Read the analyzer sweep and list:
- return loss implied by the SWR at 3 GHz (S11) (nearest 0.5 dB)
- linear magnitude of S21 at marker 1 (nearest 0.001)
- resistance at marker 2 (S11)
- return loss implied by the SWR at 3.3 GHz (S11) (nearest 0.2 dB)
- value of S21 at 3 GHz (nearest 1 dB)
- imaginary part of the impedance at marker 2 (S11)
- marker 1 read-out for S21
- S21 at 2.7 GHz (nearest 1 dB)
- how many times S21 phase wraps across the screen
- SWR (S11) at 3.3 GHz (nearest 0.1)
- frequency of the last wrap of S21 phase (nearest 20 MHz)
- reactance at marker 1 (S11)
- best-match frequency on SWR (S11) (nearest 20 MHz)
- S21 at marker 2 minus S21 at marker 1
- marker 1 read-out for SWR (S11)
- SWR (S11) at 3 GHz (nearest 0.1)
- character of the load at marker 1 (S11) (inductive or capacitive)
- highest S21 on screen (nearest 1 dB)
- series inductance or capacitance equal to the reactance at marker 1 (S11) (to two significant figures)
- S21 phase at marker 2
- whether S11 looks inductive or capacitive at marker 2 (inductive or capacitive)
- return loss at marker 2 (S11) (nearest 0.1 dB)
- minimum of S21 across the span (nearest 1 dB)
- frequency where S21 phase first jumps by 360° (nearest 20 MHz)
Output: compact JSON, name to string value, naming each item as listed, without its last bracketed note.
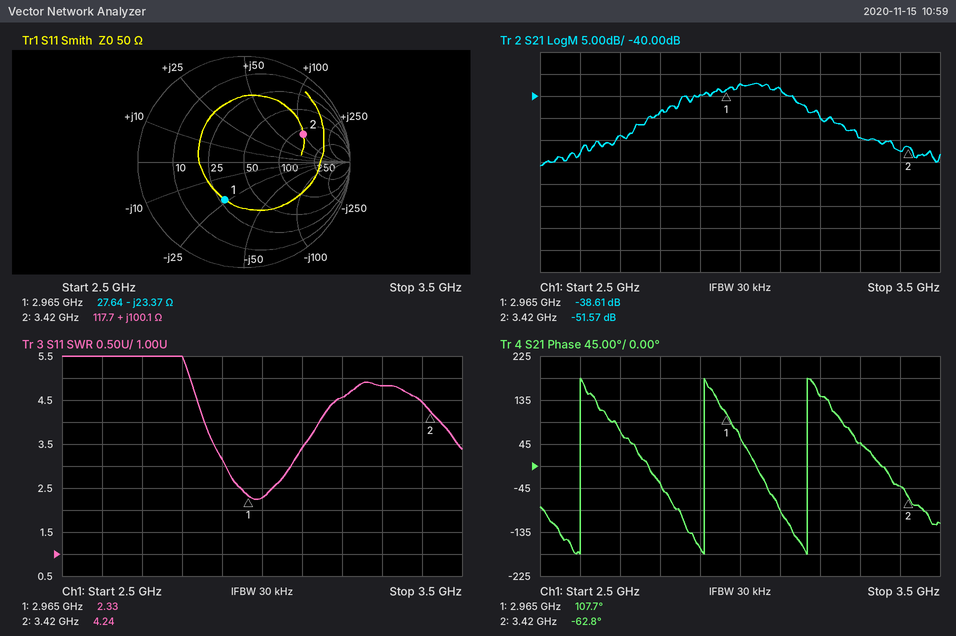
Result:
{"return loss implied by the SWR at 3 GHz (S11)": "8.0 dB", "linear magnitude of S21 at marker 1": "0.012", "resistance at marker 2": "117.7 Ω", "return loss implied by the SWR at 3.3 GHz (S11)": "3.6 dB", "value of S21 at 3 GHz": "-37 dB", "imaginary part of the impedance at marker 2": "+100.1 Ω", "marker 1 read-out for S21": "-38.61 dB", "S21 at 2.7 GHz": "-49 dB", "how many times S21 phase wraps across the screen": "3", "SWR (S11) at 3.3 GHz": "4.8", "frequency of the last wrap of S21 phase": "3.16 GHz", "reactance at marker 1": "-23.37 Ω", "best-match frequency on SWR (S11)": "2.98 GHz", "S21 at marker 2 minus S21 at marker 1": "-12.96 dB", "marker 1 read-out for SWR": "2.33", "SWR (S11) at 3 GHz": "2.3", "character of the load at marker 1 (S11)": "capacitive", "highest S21 on screen": "-37 dB", "series inductance or capacitance equal to the reactance at marker 1 (S11)": "2.3 pF", "S21 phase at marker 2": "-62.8°", "whether S11 looks inductive or capacitive at marker 2": "inductive", "return loss at marker 2 (S11)": "4.2 dB", "minimum of S21 across the span": "-56 dB", "frequency where S21 phase first jumps by 360°": "2.60 GHz"}
